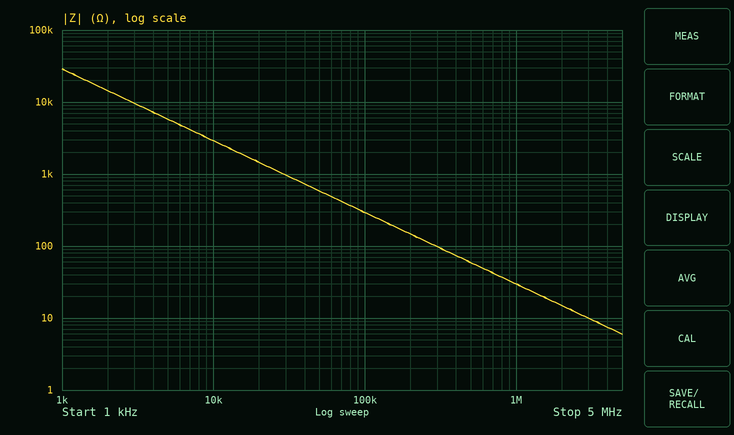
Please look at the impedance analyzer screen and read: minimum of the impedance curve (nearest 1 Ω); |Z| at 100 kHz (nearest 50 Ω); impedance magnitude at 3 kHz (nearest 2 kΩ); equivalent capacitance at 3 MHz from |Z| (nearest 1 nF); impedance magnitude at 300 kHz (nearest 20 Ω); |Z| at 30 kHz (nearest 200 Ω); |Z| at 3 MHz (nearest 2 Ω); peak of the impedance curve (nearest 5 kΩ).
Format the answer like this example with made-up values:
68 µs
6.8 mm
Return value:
6 Ω
300 Ω
10 kΩ
5 nF
100 Ω
1.0 kΩ
10 Ω
30 kΩ
